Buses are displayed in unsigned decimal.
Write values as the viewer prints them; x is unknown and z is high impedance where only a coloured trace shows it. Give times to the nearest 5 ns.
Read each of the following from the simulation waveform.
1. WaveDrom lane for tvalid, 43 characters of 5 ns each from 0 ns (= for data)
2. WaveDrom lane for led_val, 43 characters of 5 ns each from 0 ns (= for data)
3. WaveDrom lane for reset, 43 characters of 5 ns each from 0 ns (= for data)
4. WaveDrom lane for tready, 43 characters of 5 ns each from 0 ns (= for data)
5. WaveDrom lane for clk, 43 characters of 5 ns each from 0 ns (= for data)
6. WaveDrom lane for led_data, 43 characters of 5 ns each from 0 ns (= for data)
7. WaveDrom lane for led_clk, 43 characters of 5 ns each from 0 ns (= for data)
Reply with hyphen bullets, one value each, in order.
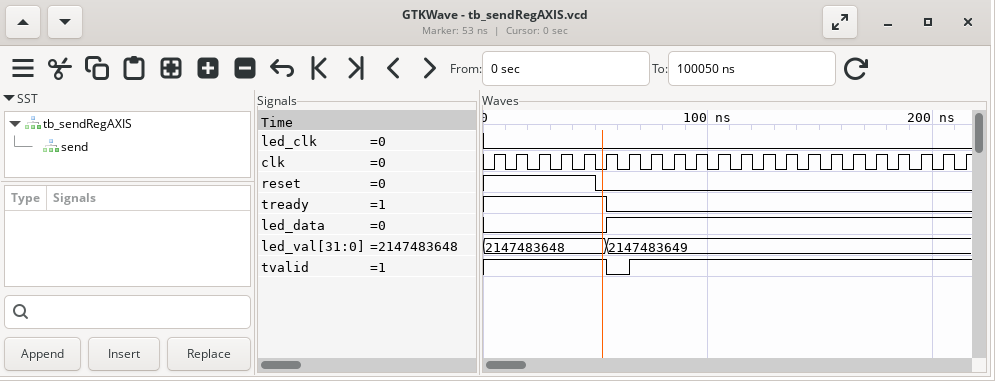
- {name: 'tvalid', wave: '1..........0.1.............................'}
- {name: 'led_val', wave: '=..........=...............................', data: '2147483648 2147483649'}
- {name: 'reset', wave: '1.........0................................'}
- {name: 'tready', wave: '1..........0...............................'}
- {name: 'clk', wave: '0101010101010101010101010101010101010101010'}
- {name: 'led_data', wave: '0..........1...............................'}
- {name: 'led_clk', wave: '0..........................................'}
